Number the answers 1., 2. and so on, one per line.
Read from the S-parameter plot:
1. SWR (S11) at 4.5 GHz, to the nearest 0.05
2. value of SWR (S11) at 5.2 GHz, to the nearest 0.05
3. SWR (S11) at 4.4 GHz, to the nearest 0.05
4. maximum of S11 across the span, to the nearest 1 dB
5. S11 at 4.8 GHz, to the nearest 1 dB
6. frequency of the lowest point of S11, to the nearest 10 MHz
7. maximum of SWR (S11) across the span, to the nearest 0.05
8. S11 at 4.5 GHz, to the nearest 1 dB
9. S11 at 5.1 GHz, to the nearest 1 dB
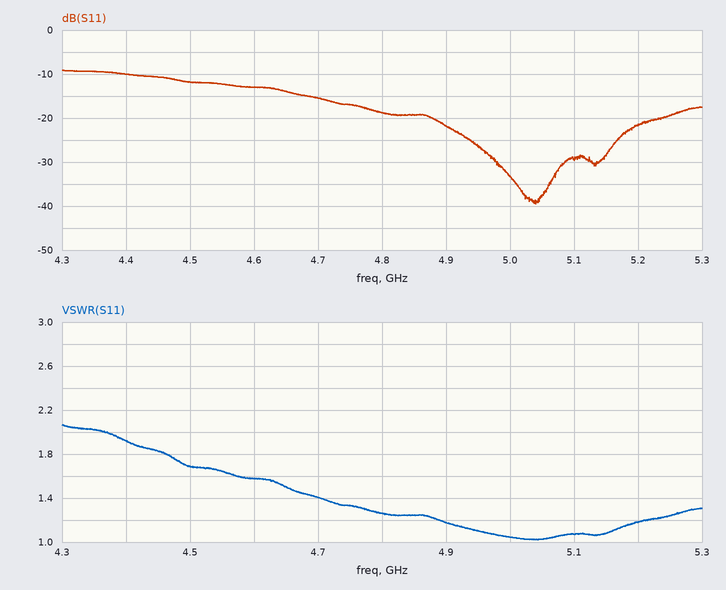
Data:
1. 1.70
2. 1.20
3. 1.90
4. -9 dB
5. -19 dB
6. 5.04 GHz
7. 2.05
8. -12 dB
9. -29 dB
